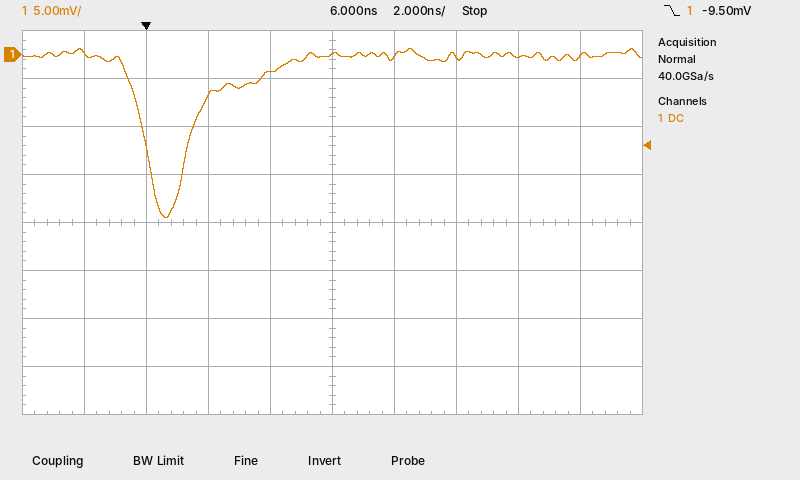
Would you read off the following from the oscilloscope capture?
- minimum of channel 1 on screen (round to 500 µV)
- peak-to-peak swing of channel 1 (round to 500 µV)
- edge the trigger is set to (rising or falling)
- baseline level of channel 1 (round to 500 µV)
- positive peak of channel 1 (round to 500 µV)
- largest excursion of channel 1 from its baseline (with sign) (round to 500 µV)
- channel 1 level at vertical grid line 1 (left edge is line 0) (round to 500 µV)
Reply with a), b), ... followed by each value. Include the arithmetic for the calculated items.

a) -17.0 mV
b) 500 µV − (-17.0 mV) = 17.5 mV
c) falling
d) 0.0 mV
e) 500 µV
f) -17.0 mV − (0.0 mV) = -17.0 mV
g) 0.0 mV
